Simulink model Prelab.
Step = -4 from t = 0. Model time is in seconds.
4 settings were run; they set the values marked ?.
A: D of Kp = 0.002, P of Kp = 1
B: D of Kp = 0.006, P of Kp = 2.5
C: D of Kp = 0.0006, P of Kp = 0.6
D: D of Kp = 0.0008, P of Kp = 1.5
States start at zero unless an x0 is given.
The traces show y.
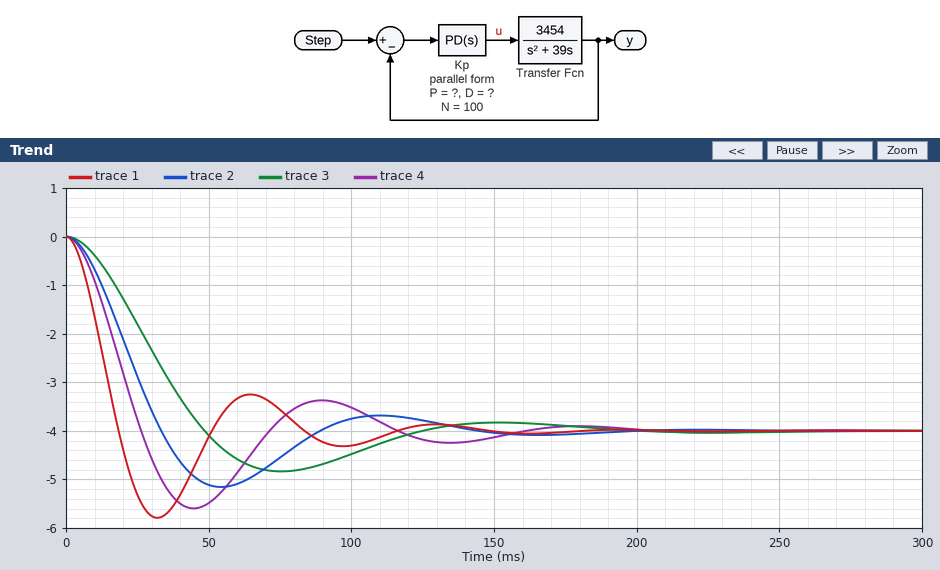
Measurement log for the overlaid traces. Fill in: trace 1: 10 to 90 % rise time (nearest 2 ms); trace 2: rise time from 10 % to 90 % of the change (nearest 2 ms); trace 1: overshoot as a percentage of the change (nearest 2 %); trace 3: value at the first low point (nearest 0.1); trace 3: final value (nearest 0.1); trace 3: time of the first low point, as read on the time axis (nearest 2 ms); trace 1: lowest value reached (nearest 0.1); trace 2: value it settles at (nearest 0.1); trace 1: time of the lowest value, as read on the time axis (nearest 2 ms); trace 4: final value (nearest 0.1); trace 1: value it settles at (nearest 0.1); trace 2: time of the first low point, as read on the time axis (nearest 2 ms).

12 ms
22 ms
44 %
-4.8
-4.0
76 ms
-5.8
-4.0
32 ms
-4.0
-4.0
54 ms
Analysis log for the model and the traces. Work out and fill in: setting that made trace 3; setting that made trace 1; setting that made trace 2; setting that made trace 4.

C
B
A
D
